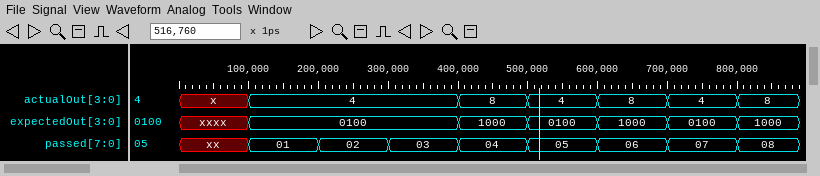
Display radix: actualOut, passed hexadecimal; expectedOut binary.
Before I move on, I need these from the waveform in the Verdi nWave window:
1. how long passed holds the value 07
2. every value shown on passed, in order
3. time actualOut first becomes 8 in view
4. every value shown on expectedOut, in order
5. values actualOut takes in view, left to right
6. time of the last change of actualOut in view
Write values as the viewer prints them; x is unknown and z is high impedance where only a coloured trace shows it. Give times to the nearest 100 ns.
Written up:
100 ns
xx, 01, 02, 03, 04, 05, 06, 07, 08
400 ns
xxxx, 0100, 1000, 0100, 1000, 0100, 1000
x, 4, 8, 4, 8, 4, 8
800 ns
